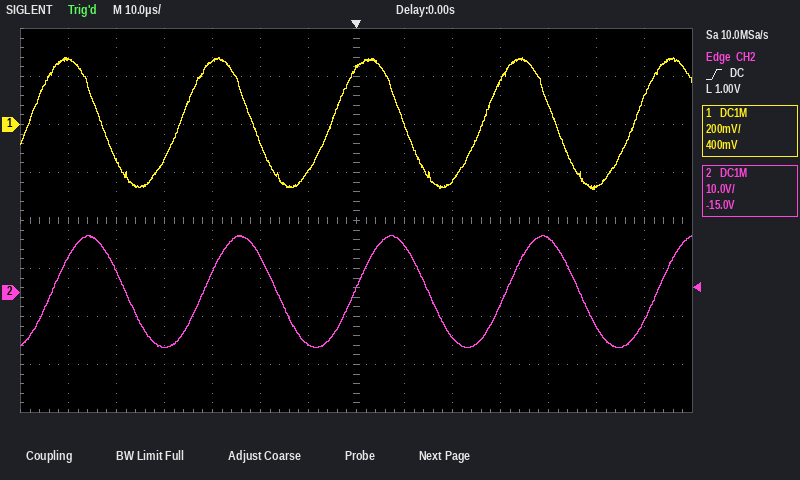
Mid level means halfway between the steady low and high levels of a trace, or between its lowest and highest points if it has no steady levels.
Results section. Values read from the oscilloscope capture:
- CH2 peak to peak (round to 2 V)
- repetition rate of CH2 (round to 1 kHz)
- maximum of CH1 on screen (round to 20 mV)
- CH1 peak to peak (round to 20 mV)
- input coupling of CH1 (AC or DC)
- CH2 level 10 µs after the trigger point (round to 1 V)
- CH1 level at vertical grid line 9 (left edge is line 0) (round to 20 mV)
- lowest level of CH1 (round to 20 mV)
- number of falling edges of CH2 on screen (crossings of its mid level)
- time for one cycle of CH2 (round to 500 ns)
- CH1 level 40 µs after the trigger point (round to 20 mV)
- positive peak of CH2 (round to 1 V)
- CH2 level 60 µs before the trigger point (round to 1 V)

24 V
32 kHz
280 mV
560 mV
DC
10 V
-240 mV
-280 mV
4
31.5 µs
80 mV
12 V
7 V
